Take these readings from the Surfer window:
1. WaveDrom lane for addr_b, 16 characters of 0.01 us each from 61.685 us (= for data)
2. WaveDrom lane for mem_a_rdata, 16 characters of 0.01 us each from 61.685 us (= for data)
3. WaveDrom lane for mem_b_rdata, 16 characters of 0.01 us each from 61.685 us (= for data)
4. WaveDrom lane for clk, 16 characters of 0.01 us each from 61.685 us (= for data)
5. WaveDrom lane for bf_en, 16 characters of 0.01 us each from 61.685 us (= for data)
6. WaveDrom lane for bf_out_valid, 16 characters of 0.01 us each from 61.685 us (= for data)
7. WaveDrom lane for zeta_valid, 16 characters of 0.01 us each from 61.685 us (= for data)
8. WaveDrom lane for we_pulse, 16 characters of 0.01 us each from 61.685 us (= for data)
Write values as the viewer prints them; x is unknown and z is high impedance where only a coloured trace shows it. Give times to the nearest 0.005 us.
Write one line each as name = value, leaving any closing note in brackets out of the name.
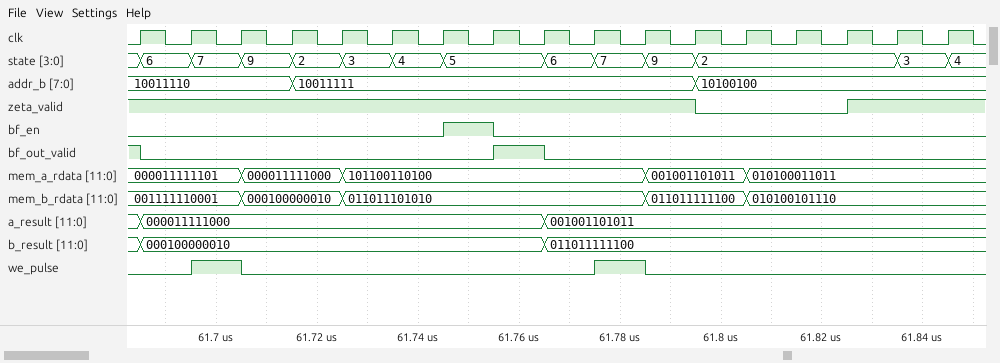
WaveDrom lane for addr_b, 16 characters of 0.01 us each from 61.685 us = {name: 'addr_b', wave: '=..=.......=....', data: '10011110 10011111 10100100'}
WaveDrom lane for mem_a_rdata, 16 characters of 0.01 us each from 61.685 us = {name: 'mem_a_rdata', wave: '=.=.=.....=.=...', data: '000011111101 000011111000 101100110100 001001101011 010100011011'}
WaveDrom lane for mem_b_rdata, 16 characters of 0.01 us each from 61.685 us = {name: 'mem_b_rdata', wave: '=.=.=.....=.=...', data: '001111110001 000100000010 011011101010 011011111100 010100101110'}
WaveDrom lane for clk, 16 characters of 0.01 us each from 61.685 us = {name: 'clk', wave: 'p...............'}
WaveDrom lane for bf_en, 16 characters of 0.01 us each from 61.685 us = {name: 'bf_en', wave: '0.....10........'}
WaveDrom lane for bf_out_valid, 16 characters of 0.01 us each from 61.685 us = {name: 'bf_out_valid', wave: '0......10.......'}
WaveDrom lane for zeta_valid, 16 characters of 0.01 us each from 61.685 us = {name: 'zeta_valid', wave: '1..........0..1.'}
WaveDrom lane for we_pulse, 16 characters of 0.01 us each from 61.685 us = {name: 'we_pulse', wave: '010......10.....'}
